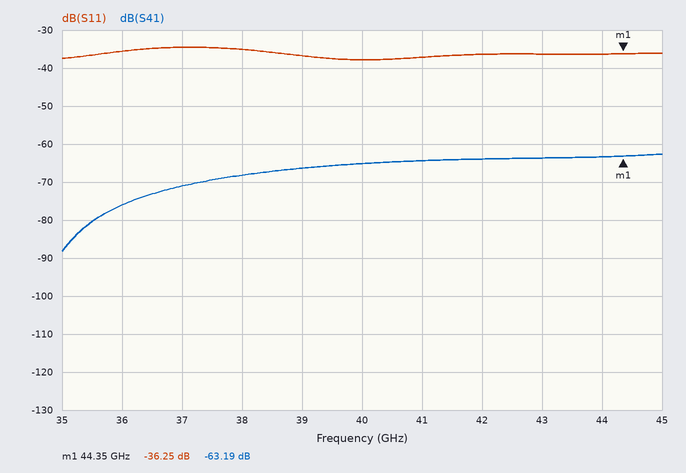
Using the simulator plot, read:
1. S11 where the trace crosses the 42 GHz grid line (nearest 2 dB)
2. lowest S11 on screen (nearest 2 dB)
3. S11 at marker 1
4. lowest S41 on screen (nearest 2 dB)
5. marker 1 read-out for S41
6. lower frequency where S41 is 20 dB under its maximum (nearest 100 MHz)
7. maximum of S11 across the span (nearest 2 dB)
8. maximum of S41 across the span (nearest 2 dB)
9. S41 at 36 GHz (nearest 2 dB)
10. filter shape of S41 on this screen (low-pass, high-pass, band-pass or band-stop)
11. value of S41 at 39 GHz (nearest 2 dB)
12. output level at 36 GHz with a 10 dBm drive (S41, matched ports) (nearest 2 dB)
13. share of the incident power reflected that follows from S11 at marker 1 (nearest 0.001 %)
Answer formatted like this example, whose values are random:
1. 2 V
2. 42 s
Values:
1. -36 dB
2. -38 dB
3. -36.25 dB
4. -88 dB
5. -63.19 dB
6. 35.3 GHz
7. -34 dB
8. -62 dB
9. -76 dB
10. high-pass
11. -66 dB
12. -66 dBm
13. 0.024 %
